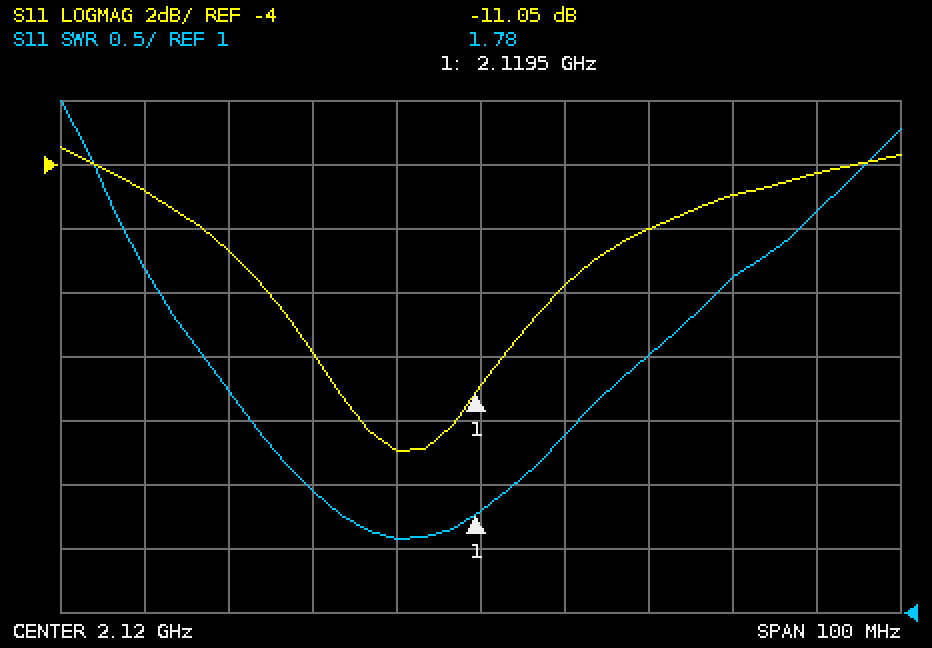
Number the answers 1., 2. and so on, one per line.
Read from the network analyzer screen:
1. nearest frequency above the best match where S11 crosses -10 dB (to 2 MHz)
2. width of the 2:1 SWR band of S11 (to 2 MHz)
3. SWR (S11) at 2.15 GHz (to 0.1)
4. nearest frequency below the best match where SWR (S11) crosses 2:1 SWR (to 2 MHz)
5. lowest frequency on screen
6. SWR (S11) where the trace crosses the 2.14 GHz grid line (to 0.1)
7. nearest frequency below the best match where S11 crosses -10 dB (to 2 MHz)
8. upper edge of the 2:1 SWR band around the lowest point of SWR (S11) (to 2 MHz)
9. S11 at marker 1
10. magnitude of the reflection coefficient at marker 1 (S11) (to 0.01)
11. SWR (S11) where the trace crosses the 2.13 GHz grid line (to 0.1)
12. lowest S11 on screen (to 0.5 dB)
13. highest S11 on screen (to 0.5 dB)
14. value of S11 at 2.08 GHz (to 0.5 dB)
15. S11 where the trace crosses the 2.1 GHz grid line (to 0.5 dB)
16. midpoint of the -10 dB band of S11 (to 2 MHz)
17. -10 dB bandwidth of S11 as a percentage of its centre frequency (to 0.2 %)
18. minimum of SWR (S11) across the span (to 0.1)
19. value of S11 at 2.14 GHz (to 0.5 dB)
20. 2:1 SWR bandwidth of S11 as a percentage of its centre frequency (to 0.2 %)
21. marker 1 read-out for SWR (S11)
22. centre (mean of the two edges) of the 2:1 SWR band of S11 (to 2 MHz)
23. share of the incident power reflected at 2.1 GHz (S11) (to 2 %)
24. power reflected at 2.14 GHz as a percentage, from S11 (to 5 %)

1. 2.122 GHz
2. 24 MHz
3. 3.6
4. 2.100 GHz
5. 2.07 GHz
6. 3.0
7. 2.100 GHz
8. 2.124 GHz
9. -11.05 dB
10. 0.28
11. 2.4
12. -13.0 dB
13. -3.5 dB
14. -5.0 dB
15. -10.0 dB
16. 2.112 GHz
17. 1.0 %
18. 1.6
19. -6.0 dB
20. 1.2 %
21. 1.78
22. 2.112 GHz
23. 10 %
24. 25 %
